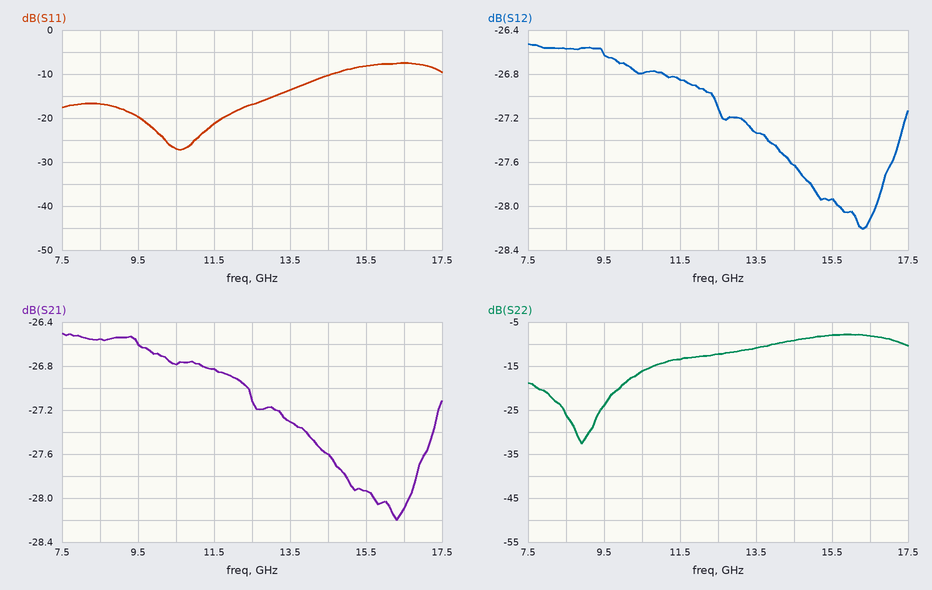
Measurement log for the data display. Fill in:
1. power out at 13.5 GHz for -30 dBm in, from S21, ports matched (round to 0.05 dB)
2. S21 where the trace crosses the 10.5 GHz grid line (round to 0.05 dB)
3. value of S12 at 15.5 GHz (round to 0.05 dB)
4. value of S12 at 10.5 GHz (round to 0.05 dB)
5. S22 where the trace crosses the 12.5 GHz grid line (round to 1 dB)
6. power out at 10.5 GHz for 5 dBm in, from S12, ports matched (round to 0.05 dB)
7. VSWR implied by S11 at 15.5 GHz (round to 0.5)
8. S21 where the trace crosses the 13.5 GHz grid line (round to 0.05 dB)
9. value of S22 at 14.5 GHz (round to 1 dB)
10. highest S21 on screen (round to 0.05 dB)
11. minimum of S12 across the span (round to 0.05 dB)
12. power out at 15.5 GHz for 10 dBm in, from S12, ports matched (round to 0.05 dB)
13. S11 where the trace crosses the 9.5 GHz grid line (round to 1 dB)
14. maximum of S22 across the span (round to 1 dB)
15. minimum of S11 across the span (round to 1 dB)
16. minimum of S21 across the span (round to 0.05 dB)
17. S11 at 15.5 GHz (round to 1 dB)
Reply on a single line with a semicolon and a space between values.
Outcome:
-57.30 dBm; -26.80 dB; -27.95 dB; -26.80 dB; -12 dB; -21.80 dBm; 2.5; -27.30 dB; -9 dB; -26.50 dB; -28.20 dB; -17.95 dBm; -20 dB; -8 dB; -27 dB; -28.20 dB; -8 dB
